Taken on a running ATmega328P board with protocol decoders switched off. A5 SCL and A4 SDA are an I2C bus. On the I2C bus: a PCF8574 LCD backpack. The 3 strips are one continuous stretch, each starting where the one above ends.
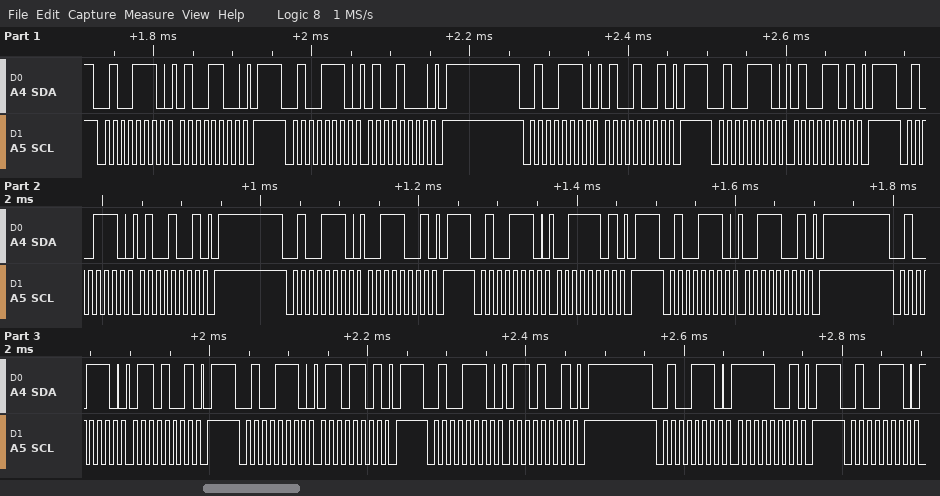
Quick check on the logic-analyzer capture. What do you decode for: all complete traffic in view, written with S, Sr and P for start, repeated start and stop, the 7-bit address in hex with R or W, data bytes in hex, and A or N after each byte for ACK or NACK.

S 27W A 4C A P S 27W A 48 A P S 27W A 49 A P S 27W A 4D A P S 27W A 49 A P S 27W A 39 A P S 27W A 3D A P S 27W A 39 A P S 27W A 69 A P S 27W A 6D A P S 27W A 69 A P S 27W A F9 A P S 27W A
